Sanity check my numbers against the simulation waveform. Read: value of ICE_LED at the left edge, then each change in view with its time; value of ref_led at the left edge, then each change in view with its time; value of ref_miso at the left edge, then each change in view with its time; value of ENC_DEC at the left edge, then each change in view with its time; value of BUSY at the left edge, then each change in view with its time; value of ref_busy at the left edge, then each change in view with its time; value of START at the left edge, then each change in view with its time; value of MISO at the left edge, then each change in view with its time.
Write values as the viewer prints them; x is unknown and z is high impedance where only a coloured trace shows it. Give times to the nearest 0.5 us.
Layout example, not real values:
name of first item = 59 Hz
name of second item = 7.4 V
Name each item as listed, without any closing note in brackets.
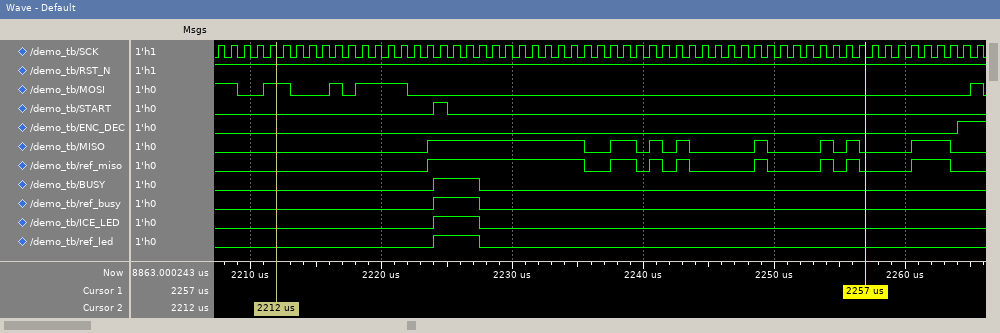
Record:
value of ICE_LED at the left edge, then each change in view with its time = 0, 1 at 2224 us, 0 at 2227.5 us
value of ref_led at the left edge, then each change in view with its time = 0, 1 at 2224 us, 0 at 2227.5 us
value of ref_miso at the left edge, then each change in view with its time = 0, 1 at 2223.5 us, 0 at 2235.5 us, 1 at 2237.5 us, 0 at 2239.5 us, 1 at 2240.5 us, 0 at 2241.5 us, 1 at 2242.5 us, 0 at 2243.5 us, 1 at 2248.5 us, 0 at 2249.5 us, 1 at 2253.5 us, 0 at 2254.5 us, 1 at 2255.5 us, 0 at 2256.5 us, 1 at 2260.5 us, 0 at 2263.5 us
value of ENC_DEC at the left edge, then each change in view with its time = 0, 1 at 2264 us
value of BUSY at the left edge, then each change in view with its time = 0, 1 at 2224 us, 0 at 2227.5 us
value of ref_busy at the left edge, then each change in view with its time = 0, 1 at 2224 us, 0 at 2227.5 us
value of START at the left edge, then each change in view with its time = 0, 1 at 2224 us, 0 at 2225 us
value of MISO at the left edge, then each change in view with its time = 0, 1 at 2223.5 us, 0 at 2235.5 us, 1 at 2237.5 us, 0 at 2239.5 us, 1 at 2240.5 us, 0 at 2241.5 us, 1 at 2242.5 us, 0 at 2243.5 us, 1 at 2248.5 us, 0 at 2249.5 us, 1 at 2253.5 us, 0 at 2254.5 us, 1 at 2255.5 us, 0 at 2256.5 us, 1 at 2260.5 us, 0 at 2263.5 us
